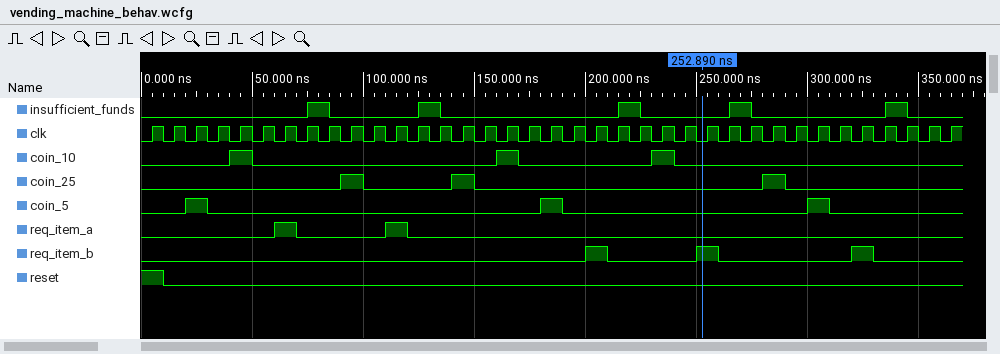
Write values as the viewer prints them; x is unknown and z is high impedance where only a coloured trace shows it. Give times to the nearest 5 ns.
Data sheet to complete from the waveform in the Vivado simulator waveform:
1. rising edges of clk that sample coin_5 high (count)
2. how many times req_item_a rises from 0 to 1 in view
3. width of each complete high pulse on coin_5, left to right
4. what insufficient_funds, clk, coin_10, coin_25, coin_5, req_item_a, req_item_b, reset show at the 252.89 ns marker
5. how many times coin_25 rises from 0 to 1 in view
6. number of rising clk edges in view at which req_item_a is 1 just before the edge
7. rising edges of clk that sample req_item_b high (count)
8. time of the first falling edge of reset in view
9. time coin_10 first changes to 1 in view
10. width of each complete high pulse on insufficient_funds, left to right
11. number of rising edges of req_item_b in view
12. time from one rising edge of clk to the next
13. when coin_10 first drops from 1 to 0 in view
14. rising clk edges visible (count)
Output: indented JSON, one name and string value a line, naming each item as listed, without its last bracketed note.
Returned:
{
  "rising edges of clk that sample coin_5 high": "3",
  "how many times req_item_a rises from 0 to 1 in view": "2",
  "width of each complete high pulse on coin_5, left to right": "10 ns, 10 ns, 10 ns",
  "what insufficient_funds, clk, coin_10, coin_25, coin_5, req_item_a, req_item_b, reset show at the 252.89 ns marker": "insufficient_funds=0, clk=0, coin_10=0, coin_25=0, coin_5=0, req_item_a=0, req_item_b=1, reset=0",
  "how many times coin_25 rises from 0 to 1 in view": "3",
  "number of rising clk edges in view at which req_item_a is 1 just before the edge": "2",
  "rising edges of clk that sample req_item_b high": "3",
  "time of the first falling edge of reset in view": "10 ns",
  "time coin_10 first changes to 1 in view": "40 ns",
  "width of each complete high pulse on insufficient_funds, left to right": "10 ns, 10 ns, 10 ns, 10 ns, 10 ns",
  "number of rising edges of req_item_b in view": "3",
  "time from one rising edge of clk to the next": "10 ns",
  "when coin_10 first drops from 1 to 0 in view": "50 ns",
  "rising clk edges visible": "37"
}
